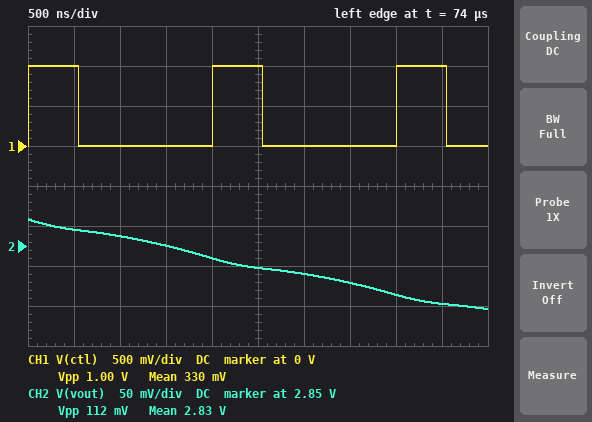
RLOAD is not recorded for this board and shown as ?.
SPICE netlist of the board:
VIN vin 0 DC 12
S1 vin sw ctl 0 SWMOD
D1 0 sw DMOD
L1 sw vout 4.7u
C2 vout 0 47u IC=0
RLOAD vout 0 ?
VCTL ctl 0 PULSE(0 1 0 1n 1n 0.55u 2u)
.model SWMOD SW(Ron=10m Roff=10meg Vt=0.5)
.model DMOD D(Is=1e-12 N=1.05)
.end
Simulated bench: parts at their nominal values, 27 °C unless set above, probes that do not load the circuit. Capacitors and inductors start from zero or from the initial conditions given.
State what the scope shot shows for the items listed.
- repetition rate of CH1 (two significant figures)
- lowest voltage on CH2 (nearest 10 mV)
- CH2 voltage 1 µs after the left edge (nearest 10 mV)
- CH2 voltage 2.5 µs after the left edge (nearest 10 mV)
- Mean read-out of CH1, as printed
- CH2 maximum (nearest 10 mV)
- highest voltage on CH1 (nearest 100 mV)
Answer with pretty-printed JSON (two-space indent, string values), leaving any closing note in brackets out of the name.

{
  "repetition rate of CH1": "500 kHz",
  "lowest voltage on CH2": "2.77 V",
  "CH2 voltage 1 µs after the left edge": "2.86 V",
  "CH2 voltage 2.5 µs after the left edge": "2.82 V",
  "Mean read-out of CH1, as printed": "330 mV",
  "CH2 maximum": "2.88 V",
  "highest voltage on CH1": "1.0 V"
}
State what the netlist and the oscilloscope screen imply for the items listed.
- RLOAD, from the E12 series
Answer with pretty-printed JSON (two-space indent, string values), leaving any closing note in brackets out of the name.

{
  "RLOAD, from the E12 series": "0.39 Ω"
}
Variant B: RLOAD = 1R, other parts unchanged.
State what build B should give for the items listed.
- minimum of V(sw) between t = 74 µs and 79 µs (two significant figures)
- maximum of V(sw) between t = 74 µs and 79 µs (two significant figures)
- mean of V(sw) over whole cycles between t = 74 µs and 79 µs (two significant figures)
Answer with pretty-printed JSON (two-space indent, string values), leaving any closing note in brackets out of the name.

{
  "minimum of V(sw) between t = 74 µs and 79 µs": "-750 mV",
  "maximum of V(sw) between t = 74 µs and 79 µs": "12 V",
  "mean of V(sw) over whole cycles between t = 74 µs and 79 µs": "2.8 V"
}
